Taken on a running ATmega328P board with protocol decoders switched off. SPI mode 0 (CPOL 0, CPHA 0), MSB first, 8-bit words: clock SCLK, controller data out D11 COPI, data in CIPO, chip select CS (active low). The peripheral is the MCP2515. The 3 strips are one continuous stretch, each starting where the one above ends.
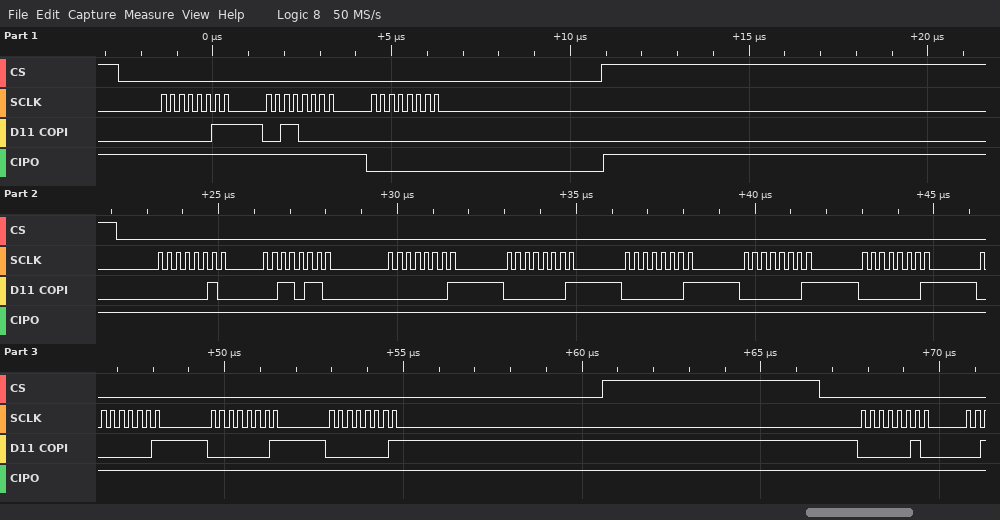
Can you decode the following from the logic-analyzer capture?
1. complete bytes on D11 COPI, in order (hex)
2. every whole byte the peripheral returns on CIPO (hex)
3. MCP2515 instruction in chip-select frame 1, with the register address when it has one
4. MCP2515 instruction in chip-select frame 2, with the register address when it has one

0x03 0x30 0x00 0x02 0x36 0x01 0x01 0x01 0x01 0x01 0x01 0x01 0x01 0x02
0xFF 0xFF 0x00 0xFF 0xFF 0xFF 0xFF 0xFF 0xFF 0xFF 0xFF 0xFF 0xFF 0xFF
READ 0x30
WRITE 0x36
